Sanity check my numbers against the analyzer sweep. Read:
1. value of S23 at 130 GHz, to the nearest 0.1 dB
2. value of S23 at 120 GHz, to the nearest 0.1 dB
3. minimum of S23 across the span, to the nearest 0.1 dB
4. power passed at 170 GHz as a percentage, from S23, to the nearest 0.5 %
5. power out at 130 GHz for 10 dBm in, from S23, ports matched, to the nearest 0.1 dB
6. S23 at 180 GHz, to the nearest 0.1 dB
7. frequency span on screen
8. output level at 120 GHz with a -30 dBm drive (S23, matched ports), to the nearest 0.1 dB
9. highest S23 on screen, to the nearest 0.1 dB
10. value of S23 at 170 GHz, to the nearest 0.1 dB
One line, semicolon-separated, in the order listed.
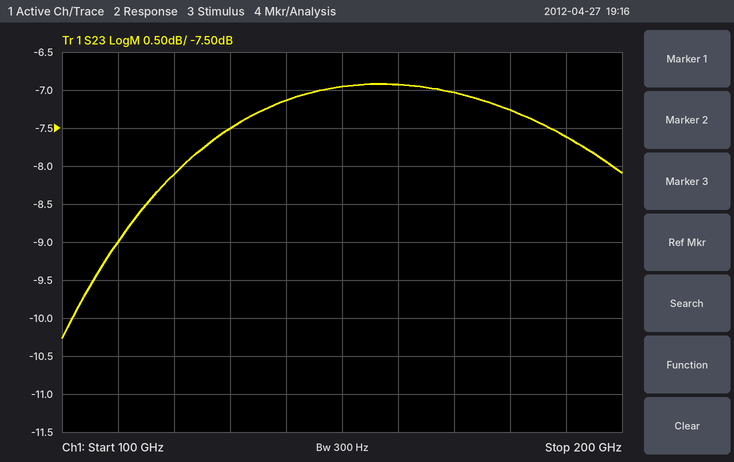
-7.5 dB; -8.1 dB; -10.3 dB; 20.0 %; 2.5 dBm; -7.3 dB; 100 GHz; -38.1 dBm; -6.9 dB; -7.0 dB
